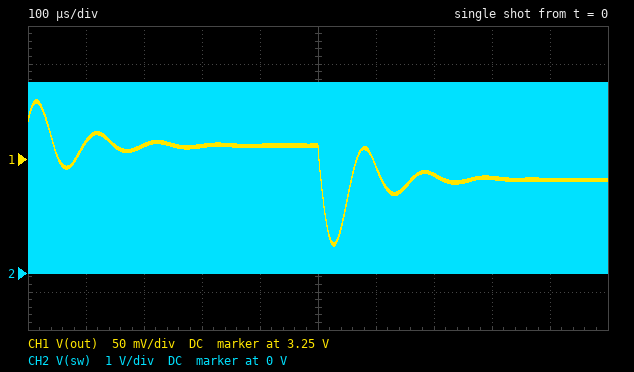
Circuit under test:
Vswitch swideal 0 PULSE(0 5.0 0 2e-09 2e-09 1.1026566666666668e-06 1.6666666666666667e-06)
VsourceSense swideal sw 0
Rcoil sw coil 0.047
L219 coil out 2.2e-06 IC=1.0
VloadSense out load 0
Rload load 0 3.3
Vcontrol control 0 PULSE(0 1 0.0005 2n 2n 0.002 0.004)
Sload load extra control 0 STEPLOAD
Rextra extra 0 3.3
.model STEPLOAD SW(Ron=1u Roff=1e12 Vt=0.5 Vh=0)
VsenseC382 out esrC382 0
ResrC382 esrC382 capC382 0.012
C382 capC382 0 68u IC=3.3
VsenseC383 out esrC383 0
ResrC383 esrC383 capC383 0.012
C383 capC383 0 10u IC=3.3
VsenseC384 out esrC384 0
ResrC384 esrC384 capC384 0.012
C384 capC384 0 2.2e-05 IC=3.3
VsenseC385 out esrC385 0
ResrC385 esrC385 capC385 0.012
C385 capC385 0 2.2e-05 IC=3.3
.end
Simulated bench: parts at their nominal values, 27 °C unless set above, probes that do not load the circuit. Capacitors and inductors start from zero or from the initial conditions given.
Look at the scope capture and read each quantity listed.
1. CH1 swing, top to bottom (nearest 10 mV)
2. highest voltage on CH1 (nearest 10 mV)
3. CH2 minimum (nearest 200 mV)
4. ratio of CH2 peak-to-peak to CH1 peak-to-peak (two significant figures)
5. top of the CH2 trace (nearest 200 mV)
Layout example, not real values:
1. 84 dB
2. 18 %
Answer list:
1. 190 mV
2. 3.33 V
3. 0 V
4. 26
5. 5.0 V
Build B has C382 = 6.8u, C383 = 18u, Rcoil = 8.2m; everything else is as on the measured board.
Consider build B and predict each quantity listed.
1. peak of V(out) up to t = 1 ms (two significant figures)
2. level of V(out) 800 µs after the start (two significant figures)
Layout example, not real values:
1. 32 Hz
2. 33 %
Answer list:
1. 3.4 V
2. 3.3 V
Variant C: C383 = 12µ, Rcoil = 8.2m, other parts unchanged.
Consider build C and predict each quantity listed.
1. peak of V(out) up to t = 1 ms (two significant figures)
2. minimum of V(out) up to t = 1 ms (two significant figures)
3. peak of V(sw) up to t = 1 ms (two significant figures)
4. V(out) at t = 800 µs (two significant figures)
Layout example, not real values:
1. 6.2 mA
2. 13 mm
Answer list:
1. 3.4 V
2. 3.2 V
3. 5.0 V
4. 3.3 V
